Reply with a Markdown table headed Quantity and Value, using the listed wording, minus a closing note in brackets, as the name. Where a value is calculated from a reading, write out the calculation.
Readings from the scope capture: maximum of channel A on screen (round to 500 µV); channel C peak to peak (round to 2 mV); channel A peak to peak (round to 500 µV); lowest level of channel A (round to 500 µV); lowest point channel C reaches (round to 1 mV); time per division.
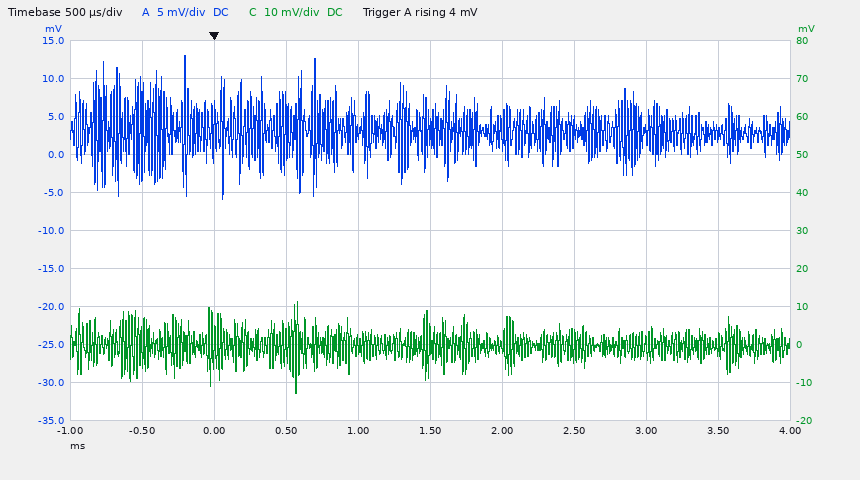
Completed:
| Quantity | Value |
|---|---|
| maximum of channel A on screen | 13.0 mV |
| channel C peak to peak | 24 mV |
| channel A peak to peak | 13.0 mV − (-6.0 mV) = 19.0 mV |
| lowest level of channel A | -6.0 mV |
| lowest point channel C reaches | -13 mV |
| time per division | 500 µs |
